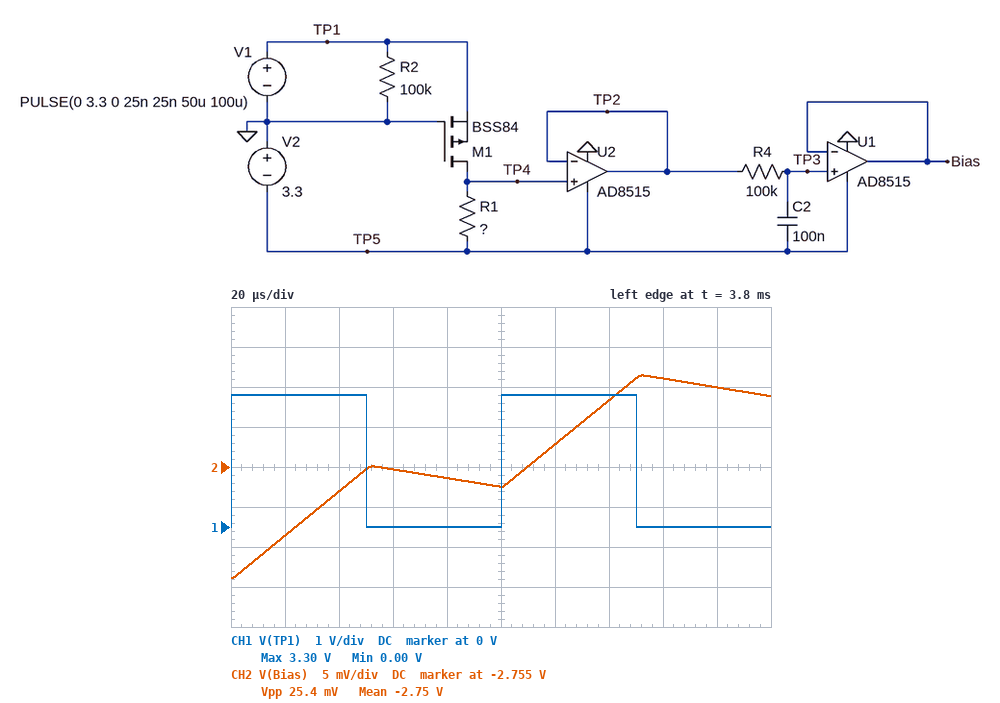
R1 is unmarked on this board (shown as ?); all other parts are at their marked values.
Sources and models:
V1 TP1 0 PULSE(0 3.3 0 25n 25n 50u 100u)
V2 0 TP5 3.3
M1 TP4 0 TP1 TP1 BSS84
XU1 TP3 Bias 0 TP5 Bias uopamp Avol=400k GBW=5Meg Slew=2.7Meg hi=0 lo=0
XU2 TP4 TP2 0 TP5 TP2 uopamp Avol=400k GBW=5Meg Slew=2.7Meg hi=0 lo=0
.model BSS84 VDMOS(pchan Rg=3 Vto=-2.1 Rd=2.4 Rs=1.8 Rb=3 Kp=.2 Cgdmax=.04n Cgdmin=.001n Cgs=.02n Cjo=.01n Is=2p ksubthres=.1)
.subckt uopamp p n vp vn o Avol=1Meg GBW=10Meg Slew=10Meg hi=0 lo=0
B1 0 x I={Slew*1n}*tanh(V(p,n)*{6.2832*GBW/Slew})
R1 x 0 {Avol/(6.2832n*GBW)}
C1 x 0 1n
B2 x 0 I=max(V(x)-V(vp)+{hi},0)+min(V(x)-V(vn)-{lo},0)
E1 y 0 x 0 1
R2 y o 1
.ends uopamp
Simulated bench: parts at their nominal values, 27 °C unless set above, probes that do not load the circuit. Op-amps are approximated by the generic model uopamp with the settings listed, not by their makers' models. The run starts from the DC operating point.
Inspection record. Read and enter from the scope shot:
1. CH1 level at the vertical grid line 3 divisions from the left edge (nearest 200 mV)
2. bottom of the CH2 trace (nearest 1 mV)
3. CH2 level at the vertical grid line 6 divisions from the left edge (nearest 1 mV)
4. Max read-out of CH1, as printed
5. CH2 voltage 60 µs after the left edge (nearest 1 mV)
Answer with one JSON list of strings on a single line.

["0 V", "-2.769 V", "-2.752 V", "3.30 V", "-2.755 V"]
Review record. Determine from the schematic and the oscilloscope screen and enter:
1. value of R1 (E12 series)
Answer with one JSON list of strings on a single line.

["68 kΩ"]
